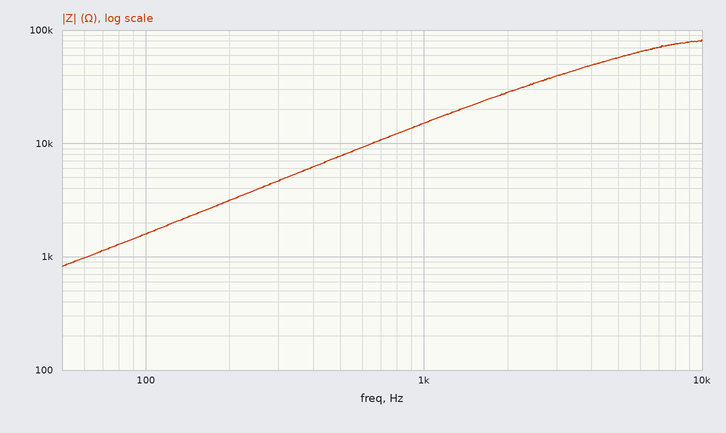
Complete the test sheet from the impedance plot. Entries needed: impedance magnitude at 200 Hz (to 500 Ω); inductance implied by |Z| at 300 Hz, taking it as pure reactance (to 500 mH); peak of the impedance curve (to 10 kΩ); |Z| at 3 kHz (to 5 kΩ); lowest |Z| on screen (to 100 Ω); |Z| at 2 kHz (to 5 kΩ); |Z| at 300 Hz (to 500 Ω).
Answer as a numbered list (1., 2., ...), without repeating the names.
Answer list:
1. 3.0 kΩ
2. 2.5 H
3. 80 kΩ
4. 40 kΩ
5. 800 Ω
6. 30 kΩ
7. 4.5 kΩ
